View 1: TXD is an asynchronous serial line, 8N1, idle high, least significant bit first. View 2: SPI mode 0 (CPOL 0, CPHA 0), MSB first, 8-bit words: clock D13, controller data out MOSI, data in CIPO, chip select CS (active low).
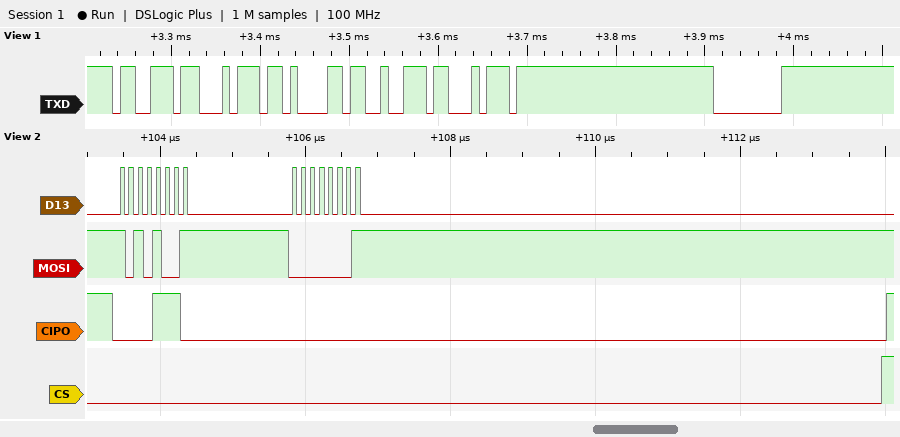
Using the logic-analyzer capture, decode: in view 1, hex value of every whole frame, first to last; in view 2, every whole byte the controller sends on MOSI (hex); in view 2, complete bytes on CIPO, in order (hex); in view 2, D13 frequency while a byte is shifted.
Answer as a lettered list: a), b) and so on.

a) 73 74 61 72 74 00
b) A9 01
c) 0E 00
d) 8 MHz
